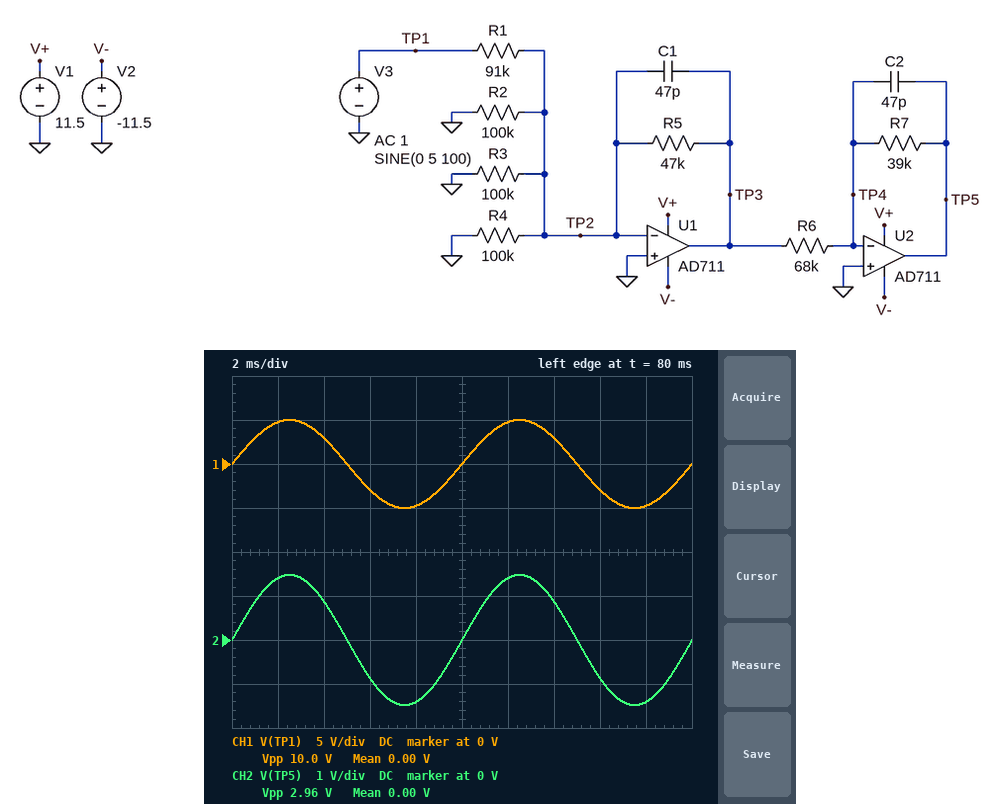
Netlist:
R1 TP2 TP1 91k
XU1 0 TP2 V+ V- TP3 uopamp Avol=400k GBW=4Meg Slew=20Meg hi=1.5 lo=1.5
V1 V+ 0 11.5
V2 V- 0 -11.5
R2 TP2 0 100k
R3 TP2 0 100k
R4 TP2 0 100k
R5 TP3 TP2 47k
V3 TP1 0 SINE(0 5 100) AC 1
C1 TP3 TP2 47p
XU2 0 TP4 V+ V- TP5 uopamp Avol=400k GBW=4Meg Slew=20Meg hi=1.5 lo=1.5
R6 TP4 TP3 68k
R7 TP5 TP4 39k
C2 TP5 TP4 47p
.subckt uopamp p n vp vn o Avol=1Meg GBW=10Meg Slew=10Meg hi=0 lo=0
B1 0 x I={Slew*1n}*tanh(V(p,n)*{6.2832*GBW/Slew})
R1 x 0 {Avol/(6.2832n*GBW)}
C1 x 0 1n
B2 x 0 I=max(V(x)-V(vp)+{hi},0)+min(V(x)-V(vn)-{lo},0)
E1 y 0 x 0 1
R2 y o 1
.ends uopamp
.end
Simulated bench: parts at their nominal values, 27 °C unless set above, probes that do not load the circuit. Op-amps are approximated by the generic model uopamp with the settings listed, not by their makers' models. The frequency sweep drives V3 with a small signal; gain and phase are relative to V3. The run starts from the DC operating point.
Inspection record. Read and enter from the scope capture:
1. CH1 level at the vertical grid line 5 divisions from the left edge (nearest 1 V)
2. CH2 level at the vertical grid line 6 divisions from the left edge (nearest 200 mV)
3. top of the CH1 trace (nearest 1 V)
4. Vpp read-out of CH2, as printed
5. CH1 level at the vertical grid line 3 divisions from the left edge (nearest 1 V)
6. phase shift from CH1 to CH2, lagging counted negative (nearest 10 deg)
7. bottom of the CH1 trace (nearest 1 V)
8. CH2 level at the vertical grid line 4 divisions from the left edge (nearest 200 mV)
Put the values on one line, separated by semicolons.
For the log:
0 V; 1.4 V; 5 V; 2.96 V; -3 V; 0 deg; -5 V; -1.4 V
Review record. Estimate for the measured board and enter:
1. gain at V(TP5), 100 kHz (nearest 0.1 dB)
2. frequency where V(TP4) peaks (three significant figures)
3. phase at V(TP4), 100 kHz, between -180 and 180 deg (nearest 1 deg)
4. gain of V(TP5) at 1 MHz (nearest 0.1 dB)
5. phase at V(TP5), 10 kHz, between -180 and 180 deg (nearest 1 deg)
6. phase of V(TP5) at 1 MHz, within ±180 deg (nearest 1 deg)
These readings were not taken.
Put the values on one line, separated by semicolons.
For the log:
-19.2 dB; 77.2 kHz; 163 deg; -55.6 dB; -15 deg; 161 deg
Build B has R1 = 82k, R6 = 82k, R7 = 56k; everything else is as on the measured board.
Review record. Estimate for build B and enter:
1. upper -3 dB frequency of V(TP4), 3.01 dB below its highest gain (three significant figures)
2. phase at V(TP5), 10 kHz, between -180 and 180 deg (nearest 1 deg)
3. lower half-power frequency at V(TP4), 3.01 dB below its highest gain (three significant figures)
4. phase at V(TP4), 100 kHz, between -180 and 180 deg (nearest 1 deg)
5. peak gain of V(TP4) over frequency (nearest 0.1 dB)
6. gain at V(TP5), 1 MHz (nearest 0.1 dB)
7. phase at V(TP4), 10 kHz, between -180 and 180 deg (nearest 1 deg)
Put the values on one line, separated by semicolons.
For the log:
156 kHz; -18 deg; 26.7 kHz; 153 deg; -50.0 dB; -56.3 dB; -108 deg
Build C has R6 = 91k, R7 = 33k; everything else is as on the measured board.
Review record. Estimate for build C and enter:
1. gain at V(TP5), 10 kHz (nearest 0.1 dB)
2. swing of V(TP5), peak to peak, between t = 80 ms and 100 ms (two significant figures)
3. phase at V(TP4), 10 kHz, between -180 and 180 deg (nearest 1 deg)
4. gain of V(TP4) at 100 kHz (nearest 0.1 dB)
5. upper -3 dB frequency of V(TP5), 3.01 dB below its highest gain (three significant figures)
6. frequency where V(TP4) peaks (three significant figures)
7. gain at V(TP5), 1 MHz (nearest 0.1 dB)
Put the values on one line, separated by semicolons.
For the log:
-14.7 dB; 1.9 V; -104 deg; -54.4 dB; 52.8 kHz; 84.0 kHz; -58.1 dB
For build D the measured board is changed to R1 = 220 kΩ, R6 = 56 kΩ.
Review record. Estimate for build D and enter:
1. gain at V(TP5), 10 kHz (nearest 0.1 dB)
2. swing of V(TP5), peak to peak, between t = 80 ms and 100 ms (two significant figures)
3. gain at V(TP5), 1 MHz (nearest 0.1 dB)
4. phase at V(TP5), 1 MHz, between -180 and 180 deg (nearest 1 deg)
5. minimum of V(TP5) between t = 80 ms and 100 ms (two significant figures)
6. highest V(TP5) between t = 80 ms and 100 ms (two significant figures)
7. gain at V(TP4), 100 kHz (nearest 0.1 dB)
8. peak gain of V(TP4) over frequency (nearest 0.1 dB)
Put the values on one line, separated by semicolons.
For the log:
-16.7 dB; 1.5 V; -61.6 dB; 161 deg; -740 mV; 740 mV; -57.2 dB; -56.9 dB
